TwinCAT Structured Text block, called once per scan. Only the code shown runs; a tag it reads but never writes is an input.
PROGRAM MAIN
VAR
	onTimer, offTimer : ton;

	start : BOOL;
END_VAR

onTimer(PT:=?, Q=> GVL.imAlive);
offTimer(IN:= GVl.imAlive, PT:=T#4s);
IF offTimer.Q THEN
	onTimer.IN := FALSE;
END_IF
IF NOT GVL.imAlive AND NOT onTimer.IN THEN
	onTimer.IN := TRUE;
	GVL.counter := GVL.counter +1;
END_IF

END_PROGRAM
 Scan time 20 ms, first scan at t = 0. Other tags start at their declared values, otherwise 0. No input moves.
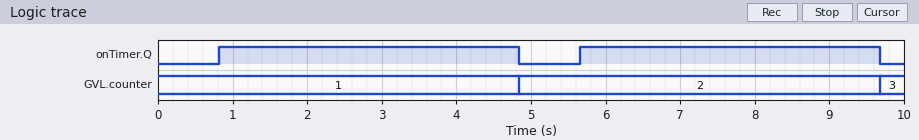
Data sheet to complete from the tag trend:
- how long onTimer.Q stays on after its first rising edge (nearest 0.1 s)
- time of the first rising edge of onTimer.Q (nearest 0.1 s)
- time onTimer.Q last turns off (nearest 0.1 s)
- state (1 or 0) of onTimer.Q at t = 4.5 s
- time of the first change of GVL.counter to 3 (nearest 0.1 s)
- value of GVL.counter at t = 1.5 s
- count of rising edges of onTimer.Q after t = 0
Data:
4.0 s
0.8 s
9.7 s
1
9.7 s
1
2
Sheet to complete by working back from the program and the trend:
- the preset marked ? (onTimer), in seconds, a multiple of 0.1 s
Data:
0.8 s
